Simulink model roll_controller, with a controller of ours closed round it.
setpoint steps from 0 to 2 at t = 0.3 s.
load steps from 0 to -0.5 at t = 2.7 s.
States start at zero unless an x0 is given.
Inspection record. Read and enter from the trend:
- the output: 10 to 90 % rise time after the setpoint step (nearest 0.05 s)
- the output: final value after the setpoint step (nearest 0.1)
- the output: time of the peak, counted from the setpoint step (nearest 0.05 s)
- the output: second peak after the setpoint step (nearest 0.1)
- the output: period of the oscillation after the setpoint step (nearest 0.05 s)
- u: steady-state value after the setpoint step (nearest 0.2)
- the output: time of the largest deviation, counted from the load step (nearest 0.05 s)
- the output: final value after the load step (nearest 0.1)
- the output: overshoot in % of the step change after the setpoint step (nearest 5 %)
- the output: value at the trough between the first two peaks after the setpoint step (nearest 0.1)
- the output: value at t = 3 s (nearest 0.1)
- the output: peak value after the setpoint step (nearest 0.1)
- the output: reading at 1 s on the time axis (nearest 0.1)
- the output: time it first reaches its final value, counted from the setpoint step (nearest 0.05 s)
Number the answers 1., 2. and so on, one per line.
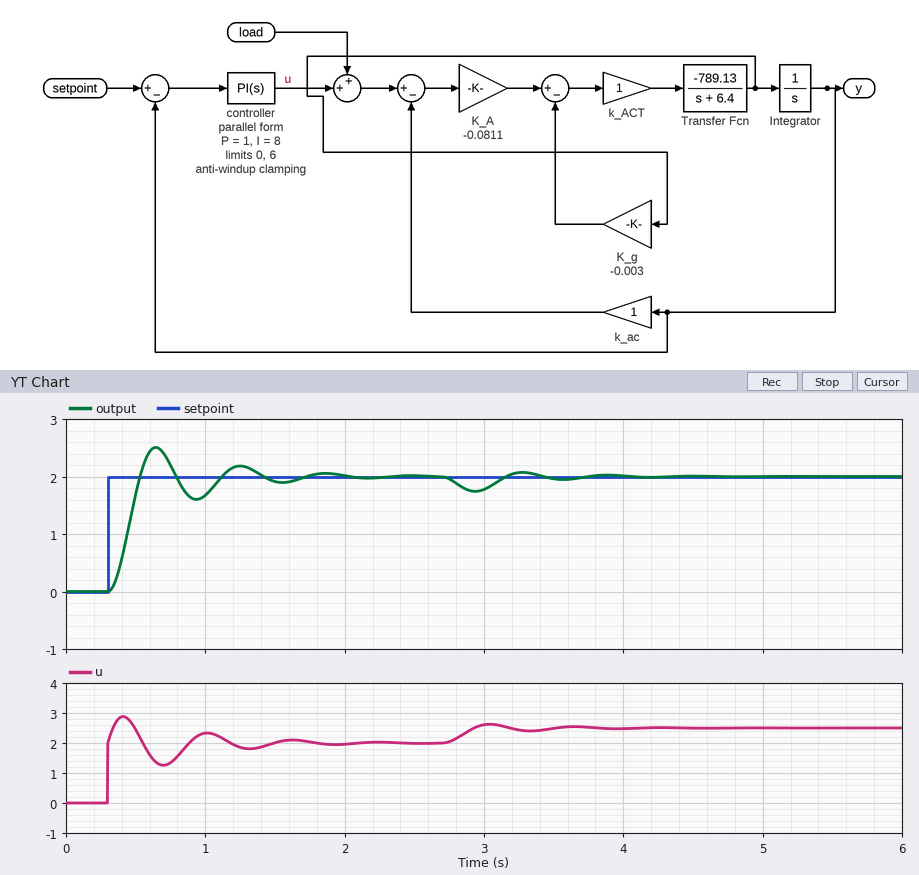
1. 0.15 s
2. 2.0
3. 0.35 s
4. 2.2
5. 0.60 s
6. 2.0
7. 0.25 s
8. 2.0
9. 25 %
10. 1.6
11. 1.8
12. 2.5
13. 1.7
14. 0.25 s
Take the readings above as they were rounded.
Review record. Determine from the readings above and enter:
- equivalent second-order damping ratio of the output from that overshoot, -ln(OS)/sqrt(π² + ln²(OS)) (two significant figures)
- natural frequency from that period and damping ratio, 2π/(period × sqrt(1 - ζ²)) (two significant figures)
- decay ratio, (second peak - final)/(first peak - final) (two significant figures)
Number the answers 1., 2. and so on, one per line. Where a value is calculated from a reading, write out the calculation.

1. ln(0.25) = -1.386; 1.386 / sqrt(9.870 + 1.922) = 0.40
2. 2π / (0.6 × sqrt(1 - 0.4²)) = 11 rad/s
3. (2.2 - 2) / (2.5 - 2) = 0.40
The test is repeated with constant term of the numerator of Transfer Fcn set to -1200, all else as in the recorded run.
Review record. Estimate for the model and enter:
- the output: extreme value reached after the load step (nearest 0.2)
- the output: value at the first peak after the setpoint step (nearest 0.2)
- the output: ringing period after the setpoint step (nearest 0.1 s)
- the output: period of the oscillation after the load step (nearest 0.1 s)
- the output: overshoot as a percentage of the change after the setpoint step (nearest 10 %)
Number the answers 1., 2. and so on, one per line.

1. 1.8
2. 2.4
3. 0.5 s
4. 0.5 s
5. 20 %
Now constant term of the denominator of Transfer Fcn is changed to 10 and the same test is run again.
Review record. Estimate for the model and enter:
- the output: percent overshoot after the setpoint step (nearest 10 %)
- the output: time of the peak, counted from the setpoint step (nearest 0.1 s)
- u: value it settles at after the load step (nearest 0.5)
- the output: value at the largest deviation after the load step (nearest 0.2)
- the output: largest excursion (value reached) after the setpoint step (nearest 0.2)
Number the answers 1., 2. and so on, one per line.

1. 20 %
2. 0.4 s
3. 2.5
4. 1.8
5. 2.4
